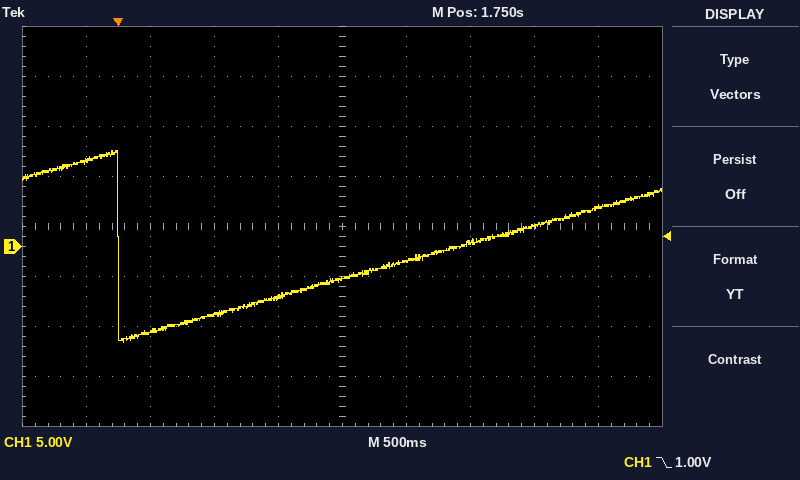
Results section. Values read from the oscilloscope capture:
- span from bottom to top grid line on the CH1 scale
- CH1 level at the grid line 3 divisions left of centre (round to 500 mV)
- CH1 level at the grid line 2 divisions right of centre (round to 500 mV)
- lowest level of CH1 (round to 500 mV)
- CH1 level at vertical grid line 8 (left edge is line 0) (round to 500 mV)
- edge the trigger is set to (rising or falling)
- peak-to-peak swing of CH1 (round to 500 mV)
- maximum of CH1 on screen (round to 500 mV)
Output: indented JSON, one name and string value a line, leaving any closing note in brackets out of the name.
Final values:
{
  "span from bottom to top grid line on the CH1 scale": "40 V",
  "CH1 level at the grid line 3 divisions left of centre": "-8.5 V",
  "CH1 level at the grid line 2 divisions right of centre": "500 mV",
  "lowest level of CH1": "-9.5 V",
  "CH1 level at vertical grid line 8 (left edge is line 0)": "2.0 V",
  "edge the trigger is set to": "falling",
  "peak-to-peak swing of CH1": "19.0 V",
  "maximum of CH1 on screen": "9.5 V"
}
